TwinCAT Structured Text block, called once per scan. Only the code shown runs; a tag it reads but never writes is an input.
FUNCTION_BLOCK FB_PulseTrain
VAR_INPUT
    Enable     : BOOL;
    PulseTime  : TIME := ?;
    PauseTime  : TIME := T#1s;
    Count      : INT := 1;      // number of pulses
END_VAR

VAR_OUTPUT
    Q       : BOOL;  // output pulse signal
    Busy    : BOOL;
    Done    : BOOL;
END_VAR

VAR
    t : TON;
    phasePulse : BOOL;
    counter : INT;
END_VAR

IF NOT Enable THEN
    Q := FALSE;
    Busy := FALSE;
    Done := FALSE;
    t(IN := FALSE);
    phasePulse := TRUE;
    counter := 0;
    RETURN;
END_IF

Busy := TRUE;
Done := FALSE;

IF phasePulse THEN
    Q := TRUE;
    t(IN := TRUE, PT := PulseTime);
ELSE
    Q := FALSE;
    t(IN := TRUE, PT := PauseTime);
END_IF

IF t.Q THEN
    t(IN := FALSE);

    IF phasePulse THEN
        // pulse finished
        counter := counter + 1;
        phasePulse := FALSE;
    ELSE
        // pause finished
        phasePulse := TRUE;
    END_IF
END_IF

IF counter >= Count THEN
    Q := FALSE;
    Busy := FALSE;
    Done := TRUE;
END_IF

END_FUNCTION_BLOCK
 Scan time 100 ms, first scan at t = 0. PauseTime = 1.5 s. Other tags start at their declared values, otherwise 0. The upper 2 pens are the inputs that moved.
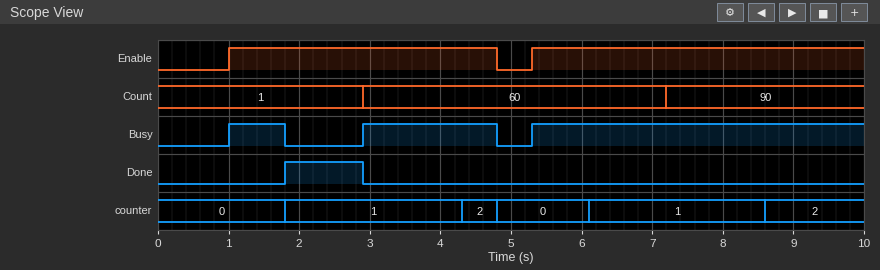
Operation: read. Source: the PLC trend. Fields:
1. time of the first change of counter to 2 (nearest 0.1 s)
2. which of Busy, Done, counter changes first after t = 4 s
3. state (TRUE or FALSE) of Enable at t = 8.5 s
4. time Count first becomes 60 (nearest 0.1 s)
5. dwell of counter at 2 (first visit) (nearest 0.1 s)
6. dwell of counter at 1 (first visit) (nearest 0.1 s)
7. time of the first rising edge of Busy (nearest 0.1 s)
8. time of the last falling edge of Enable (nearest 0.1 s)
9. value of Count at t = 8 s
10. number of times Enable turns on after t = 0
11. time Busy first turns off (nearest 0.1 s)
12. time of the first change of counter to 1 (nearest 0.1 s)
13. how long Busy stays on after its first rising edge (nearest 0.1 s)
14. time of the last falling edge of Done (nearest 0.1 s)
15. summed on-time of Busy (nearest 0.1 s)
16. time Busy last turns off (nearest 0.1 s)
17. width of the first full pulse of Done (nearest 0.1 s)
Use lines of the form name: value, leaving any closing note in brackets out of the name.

time of the first change of counter to 2: 4.3 s
which of Busy, Done, counter changes first after t = 4 s: counter
state (TRUE or FALSE) of Enable at t = 8.5 s: TRUE
time Count first becomes 60: 2.9 s
dwell of counter at 2 (first visit): 0.5 s
dwell of counter at 1 (first visit): 2.5 s
time of the first rising edge of Busy: 1.0 s
time of the last falling edge of Enable: 4.8 s
value of Count at t = 8 s: 90
number of times Enable turns on after t = 0: 2
time Busy first turns off: 1.8 s
time of the first change of counter to 1: 1.8 s
how long Busy stays on after its first rising edge: 0.8 s
time of the last falling edge of Done: 2.9 s
summed on-time of Busy: 7.4 s
time Busy last turns off: 4.8 s
width of the first full pulse of Done: 1.1 s
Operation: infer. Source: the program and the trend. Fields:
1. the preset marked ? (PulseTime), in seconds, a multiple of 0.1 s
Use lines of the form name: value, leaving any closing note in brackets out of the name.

the preset marked ? (PulseTime), in seconds, a multiple of 0.1 s: 0.8 s
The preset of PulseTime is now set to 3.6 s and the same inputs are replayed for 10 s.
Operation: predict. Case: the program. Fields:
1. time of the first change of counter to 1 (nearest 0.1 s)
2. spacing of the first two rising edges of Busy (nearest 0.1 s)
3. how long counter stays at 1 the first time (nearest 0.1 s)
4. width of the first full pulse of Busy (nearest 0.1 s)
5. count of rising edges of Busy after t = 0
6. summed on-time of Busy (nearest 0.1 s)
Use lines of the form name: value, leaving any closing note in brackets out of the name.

time of the first change of counter to 1: 4.6 s
spacing of the first two rising edges of Busy: 4.3 s
how long counter stays at 1 the first time: 0.2 s
width of the first full pulse of Busy: 3.8 s
count of rising edges of Busy after t = 0: 2
summed on-time of Busy: 8.5 s
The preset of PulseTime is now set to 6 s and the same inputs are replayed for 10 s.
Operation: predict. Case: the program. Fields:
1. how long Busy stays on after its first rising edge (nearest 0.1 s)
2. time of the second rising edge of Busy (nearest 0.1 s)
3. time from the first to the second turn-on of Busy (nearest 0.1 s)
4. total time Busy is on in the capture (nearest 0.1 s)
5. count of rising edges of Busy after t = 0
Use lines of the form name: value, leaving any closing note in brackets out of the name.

how long Busy stays on after its first rising edge: 3.8 s
time of the second rising edge of Busy: 5.3 s
time from the first to the second turn-on of Busy: 4.3 s
total time Busy is on in the capture: 8.5 s
count of rising edges of Busy after t = 0: 2
